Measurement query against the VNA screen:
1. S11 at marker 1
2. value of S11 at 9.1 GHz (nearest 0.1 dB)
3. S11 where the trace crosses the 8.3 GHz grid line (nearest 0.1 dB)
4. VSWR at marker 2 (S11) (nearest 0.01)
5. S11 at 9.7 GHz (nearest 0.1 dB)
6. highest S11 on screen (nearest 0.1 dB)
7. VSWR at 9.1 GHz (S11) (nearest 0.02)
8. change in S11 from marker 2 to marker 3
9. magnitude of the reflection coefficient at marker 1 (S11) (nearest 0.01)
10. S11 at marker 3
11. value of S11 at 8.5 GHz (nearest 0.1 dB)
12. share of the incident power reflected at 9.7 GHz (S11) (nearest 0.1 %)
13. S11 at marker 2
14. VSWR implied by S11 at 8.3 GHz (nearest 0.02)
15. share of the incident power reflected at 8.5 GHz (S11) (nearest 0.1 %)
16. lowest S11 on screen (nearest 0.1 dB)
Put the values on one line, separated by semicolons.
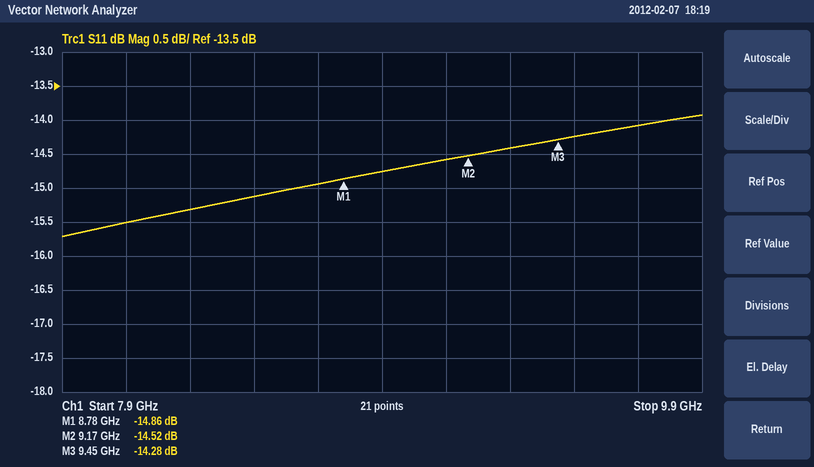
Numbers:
-14.86 dB; -14.6 dB; -15.3 dB; 1.46; -14.1 dB; -13.9 dB; 1.46; 0.24 dB; 0.18; -14.28 dB; -15.1 dB; 3.9 %; -14.52 dB; 1.42; 3.1 %; -15.7 dB
